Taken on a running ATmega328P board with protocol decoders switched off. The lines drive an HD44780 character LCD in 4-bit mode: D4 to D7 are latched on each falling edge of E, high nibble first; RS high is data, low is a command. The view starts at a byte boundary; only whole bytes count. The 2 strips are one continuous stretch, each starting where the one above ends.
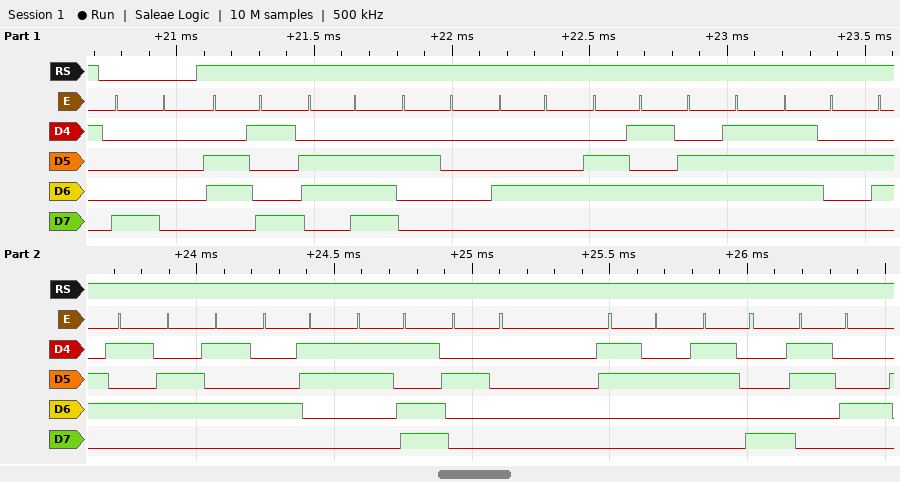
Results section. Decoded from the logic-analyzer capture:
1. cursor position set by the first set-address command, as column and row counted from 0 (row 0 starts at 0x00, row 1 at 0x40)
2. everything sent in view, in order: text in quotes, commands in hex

column 0, row 0
0x80 "in DegreeC= 284"
